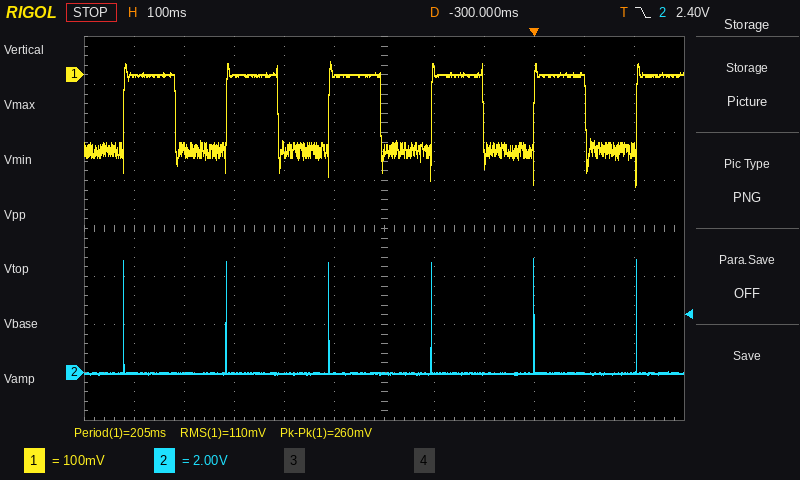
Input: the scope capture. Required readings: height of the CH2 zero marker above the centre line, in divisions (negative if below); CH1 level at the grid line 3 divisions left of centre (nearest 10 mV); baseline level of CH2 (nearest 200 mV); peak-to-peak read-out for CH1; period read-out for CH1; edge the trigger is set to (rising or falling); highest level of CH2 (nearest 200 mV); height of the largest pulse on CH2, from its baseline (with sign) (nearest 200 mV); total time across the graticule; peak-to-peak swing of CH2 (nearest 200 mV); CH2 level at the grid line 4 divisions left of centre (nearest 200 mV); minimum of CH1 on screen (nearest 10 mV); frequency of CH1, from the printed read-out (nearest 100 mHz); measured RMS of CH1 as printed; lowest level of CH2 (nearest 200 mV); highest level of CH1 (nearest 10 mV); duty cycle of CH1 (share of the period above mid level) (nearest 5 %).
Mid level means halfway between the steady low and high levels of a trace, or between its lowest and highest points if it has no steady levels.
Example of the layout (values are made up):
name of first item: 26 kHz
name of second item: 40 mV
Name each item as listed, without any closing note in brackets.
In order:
height of the CH2 zero marker above the centre line, in divisions: -3.0 div
CH1 level at the grid line 3 divisions left of centre: 0 mV
baseline level of CH2: 0.0 V
peak-to-peak read-out for CH1: 260 mV
period read-out for CH1: 205 ms
edge the trigger is set to: falling
highest level of CH2: 4.8 V
height of the largest pulse on CH2, from its baseline (with sign): +4.8 V
total time across the graticule: 1.2 s
peak-to-peak swing of CH2: 4.8 V
CH2 level at the grid line 4 divisions left of centre: 0.0 V
minimum of CH1 on screen: -230 mV
frequency of CH1, from the printed read-out: 4.9 Hz
measured RMS of CH1 as printed: 110 mV
lowest level of CH2: 0.0 V
highest level of CH1: 30 mV
duty cycle of CH1 (share of the period above mid level): 50 %
